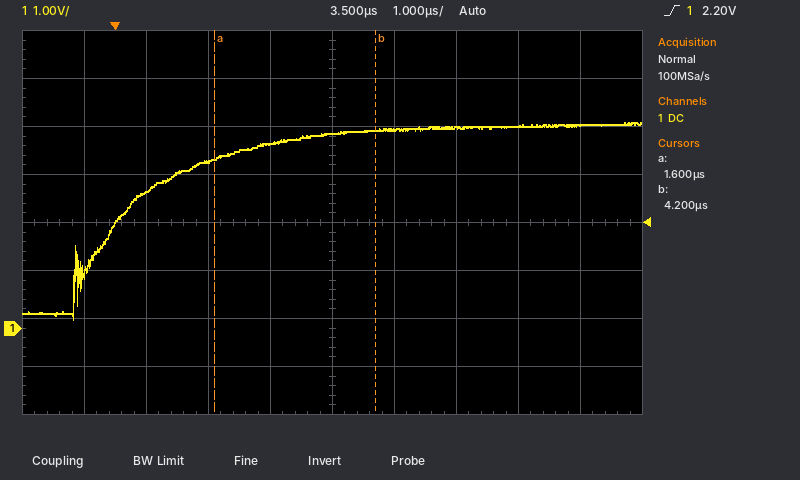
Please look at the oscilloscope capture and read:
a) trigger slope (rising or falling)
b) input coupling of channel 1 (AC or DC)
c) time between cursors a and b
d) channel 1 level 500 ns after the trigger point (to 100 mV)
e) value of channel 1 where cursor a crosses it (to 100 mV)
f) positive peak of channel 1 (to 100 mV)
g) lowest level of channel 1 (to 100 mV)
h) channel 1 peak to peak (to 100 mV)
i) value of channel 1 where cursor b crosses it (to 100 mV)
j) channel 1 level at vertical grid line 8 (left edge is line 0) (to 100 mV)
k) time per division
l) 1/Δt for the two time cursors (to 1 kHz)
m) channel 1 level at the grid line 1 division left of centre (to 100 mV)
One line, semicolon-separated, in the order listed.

rising; DC; 2.6 µs; 2.8 V; 3.5 V; 4.3 V; 200 mV; 4.1 V; 4.1 V; 4.2 V; 1 µs; 385 kHz; 3.8 V
